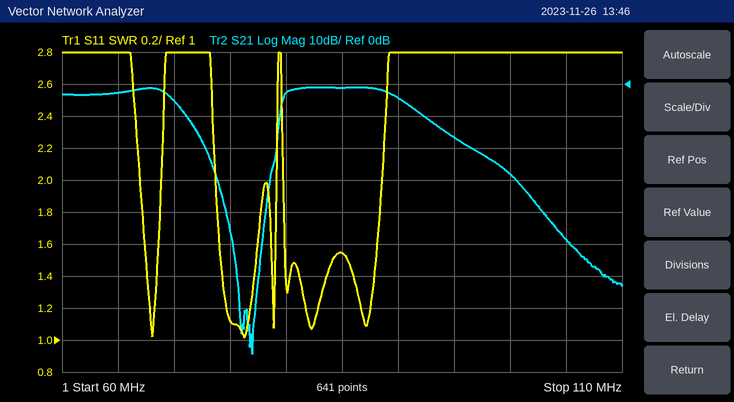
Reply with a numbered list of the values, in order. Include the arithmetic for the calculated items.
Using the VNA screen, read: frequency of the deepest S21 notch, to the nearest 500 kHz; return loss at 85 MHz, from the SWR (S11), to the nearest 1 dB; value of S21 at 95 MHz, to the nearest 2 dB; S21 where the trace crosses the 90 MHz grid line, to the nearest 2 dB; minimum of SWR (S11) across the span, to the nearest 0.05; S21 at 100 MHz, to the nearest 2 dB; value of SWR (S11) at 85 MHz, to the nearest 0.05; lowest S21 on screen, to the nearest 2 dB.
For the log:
1. 77.0 MHz
2. −20 log10((1.55 − 1)/(1.55 + 1)) ≈ 13 dB
3. -16 dB
4. -4 dB
5. 1.00
6. -28 dB
7. 1.55
8. -84 dB
